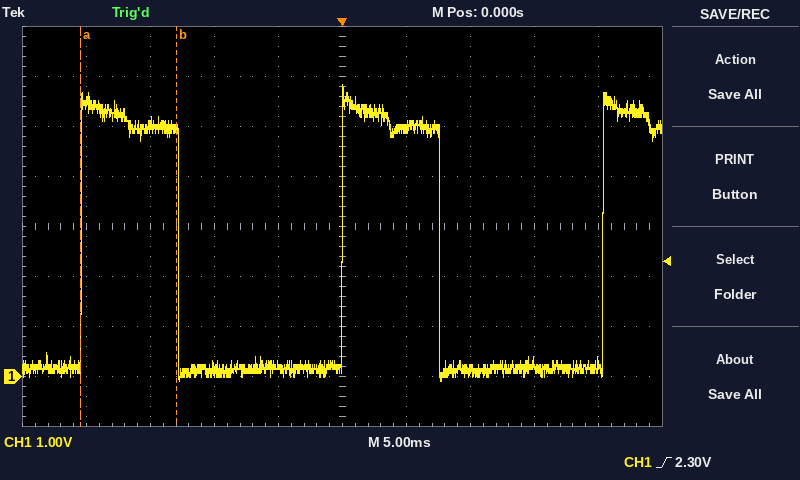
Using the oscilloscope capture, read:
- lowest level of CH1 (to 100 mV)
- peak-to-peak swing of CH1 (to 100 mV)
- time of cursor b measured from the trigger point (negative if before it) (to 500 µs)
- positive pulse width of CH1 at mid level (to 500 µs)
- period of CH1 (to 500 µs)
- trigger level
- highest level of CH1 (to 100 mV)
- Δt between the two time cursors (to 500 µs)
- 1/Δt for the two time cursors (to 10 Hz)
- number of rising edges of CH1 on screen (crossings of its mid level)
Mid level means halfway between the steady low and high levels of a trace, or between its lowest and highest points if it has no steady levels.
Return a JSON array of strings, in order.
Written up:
["-100 mV", "5.9 V", "-13.0 ms", "7.5 ms", "20.5 ms", "2.30 V", "5.8 V", "7.5 ms", "130 Hz", "3"]
